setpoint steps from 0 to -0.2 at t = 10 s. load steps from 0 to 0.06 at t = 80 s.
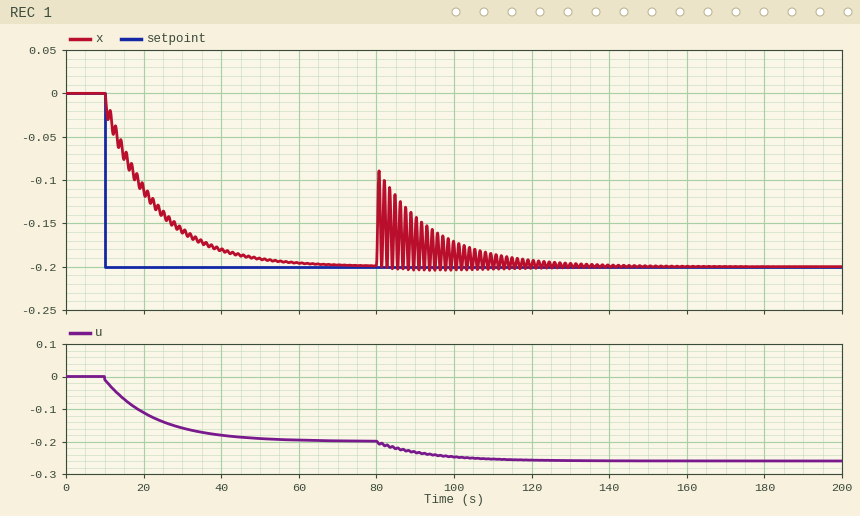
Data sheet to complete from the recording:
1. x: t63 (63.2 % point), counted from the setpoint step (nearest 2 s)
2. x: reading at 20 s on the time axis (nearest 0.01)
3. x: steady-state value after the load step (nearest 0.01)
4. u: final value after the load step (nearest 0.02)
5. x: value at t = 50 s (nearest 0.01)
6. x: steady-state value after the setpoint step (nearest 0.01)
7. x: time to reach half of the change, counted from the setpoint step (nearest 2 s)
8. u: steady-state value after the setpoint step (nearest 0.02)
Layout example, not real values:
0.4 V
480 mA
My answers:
12 s
-0.11
-0.20
-0.26
-0.19
-0.20
8 s
-0.20
